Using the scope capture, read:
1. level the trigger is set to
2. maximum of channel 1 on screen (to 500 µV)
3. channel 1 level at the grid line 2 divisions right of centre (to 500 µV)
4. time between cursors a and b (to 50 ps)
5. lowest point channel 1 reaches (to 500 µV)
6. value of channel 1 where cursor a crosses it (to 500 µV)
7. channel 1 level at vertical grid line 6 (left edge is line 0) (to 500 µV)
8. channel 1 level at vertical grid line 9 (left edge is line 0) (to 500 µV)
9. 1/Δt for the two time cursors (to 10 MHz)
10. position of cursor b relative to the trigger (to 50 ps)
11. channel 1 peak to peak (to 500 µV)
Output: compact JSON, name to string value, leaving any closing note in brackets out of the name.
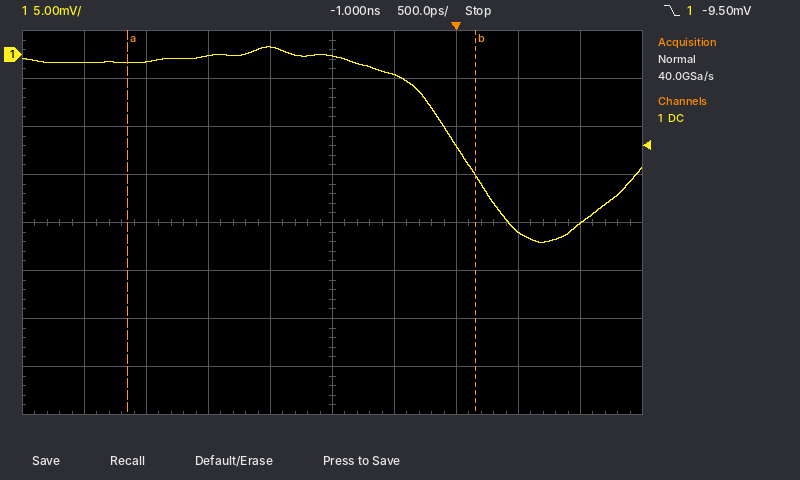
{"level the trigger is set to": "-9.50 mV", "maximum of channel 1 on screen": "1.0 mV", "channel 1 level at the grid line 2 divisions right of centre": "-9.5 mV", "time between cursors a and b": "2.80 ns", "lowest point channel 1 reaches": "-19.5 mV", "value of channel 1 where cursor a crosses it": "-1.0 mV", "channel 1 level at vertical grid line 6 (left edge is line 0)": "-2.0 mV", "channel 1 level at vertical grid line 9 (left edge is line 0)": "-17.5 mV", "1/Δt for the two time cursors": "360 MHz", "position of cursor b relative to the trigger": "+150 ps", "channel 1 peak to peak": "20.5 mV"}
